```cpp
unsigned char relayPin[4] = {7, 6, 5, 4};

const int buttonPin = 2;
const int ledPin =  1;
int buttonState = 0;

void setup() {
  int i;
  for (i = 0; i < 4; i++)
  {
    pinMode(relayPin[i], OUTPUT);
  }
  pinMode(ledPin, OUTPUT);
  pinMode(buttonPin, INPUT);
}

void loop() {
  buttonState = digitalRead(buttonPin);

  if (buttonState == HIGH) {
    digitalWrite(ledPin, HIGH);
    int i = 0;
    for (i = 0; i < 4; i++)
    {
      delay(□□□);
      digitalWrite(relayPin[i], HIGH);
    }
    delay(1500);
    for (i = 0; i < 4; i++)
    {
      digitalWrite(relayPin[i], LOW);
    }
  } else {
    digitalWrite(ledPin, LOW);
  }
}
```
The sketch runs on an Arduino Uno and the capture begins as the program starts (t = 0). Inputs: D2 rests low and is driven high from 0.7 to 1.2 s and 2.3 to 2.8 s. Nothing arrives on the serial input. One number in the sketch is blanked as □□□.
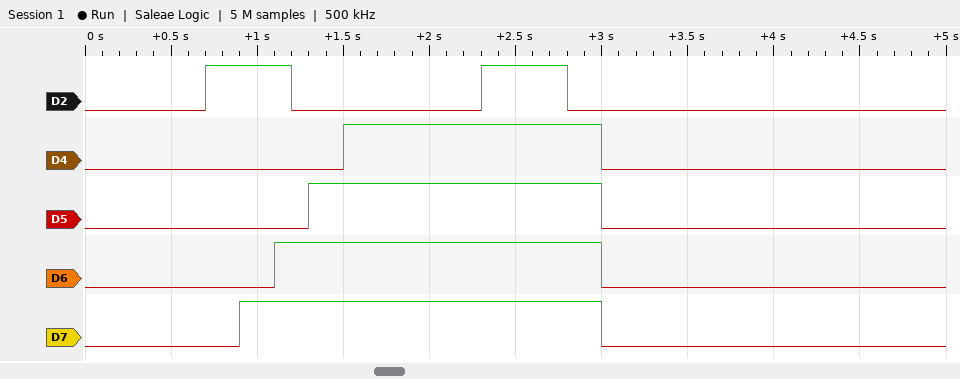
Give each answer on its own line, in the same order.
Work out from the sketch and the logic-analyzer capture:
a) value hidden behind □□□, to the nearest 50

200
